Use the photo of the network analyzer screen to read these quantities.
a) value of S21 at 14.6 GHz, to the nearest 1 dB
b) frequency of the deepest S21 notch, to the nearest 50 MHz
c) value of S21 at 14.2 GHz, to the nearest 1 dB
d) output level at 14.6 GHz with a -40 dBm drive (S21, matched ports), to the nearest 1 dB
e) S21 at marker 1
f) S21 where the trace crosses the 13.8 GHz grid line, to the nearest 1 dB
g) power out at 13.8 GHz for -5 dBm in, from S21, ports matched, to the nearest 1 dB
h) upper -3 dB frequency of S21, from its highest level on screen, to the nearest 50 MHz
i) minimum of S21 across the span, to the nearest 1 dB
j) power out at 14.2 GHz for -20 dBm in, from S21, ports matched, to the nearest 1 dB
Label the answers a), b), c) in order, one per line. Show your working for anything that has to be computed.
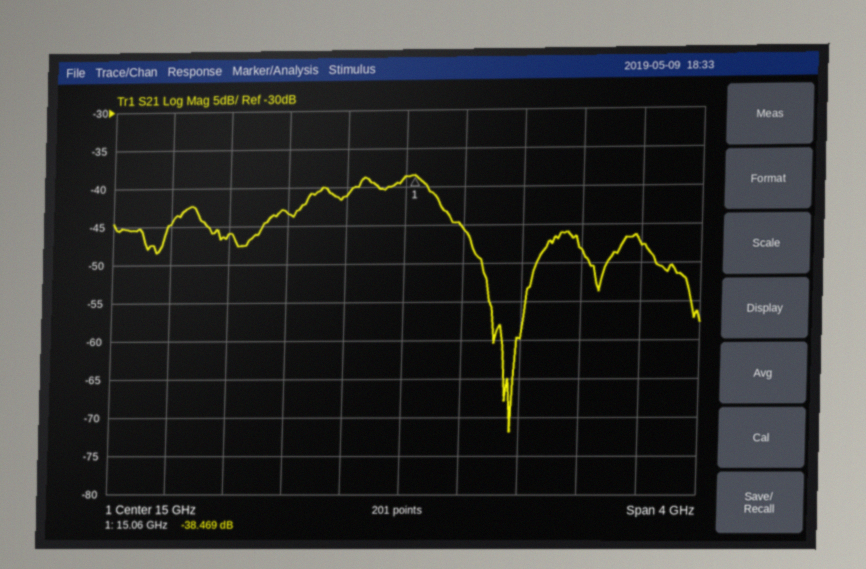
a) -41 dB
b) 15.75 GHz
c) -43 dB
d) -40 dBm + (-41 dB) = -81 dBm
e) -38.469 dB
f) -46 dB
g) -5 dBm + (-46 dB) = -51 dBm
h) 15.20 GHz
i) -72 dB
j) -20 dBm + (-43 dB) = -63 dBm
